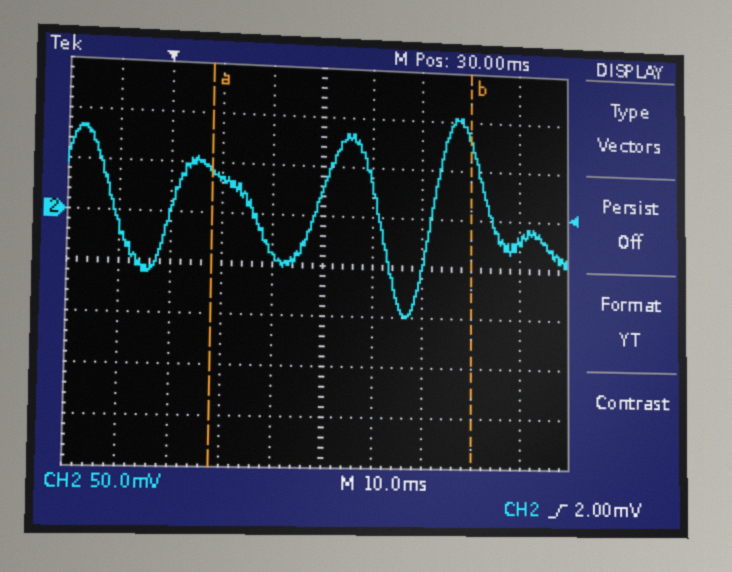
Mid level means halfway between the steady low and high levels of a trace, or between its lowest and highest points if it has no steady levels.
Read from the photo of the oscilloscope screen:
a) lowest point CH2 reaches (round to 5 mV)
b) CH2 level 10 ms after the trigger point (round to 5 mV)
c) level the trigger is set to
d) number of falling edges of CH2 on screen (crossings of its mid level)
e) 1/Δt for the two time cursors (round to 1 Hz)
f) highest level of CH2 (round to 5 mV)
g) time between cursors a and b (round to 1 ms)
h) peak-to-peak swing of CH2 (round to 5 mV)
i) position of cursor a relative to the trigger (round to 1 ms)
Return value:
-100 mV
35 mV
2.00 mV
4
19 Hz
105 mV
52 ms
205 mV
+8 ms
